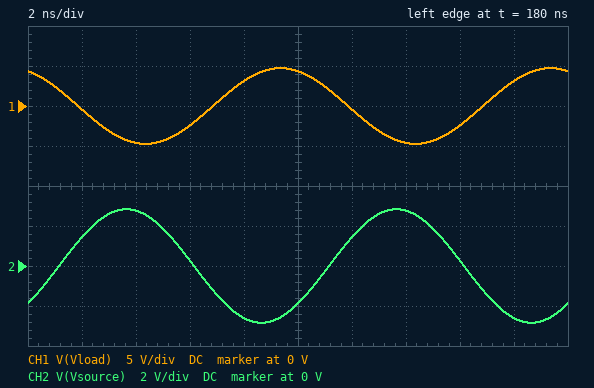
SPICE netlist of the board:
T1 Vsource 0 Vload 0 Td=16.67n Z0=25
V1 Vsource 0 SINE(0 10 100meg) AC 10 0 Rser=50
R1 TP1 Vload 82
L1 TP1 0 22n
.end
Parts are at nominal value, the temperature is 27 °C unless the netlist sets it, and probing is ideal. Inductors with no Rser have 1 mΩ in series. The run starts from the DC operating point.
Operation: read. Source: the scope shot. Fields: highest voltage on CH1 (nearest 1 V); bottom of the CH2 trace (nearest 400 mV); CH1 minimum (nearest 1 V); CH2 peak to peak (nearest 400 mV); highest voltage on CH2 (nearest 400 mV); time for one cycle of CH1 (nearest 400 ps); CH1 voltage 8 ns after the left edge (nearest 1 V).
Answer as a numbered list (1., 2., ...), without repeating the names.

1. 5 V
2. -2.8 V
3. -5 V
4. 5.6 V
5. 2.8 V
6. 10.0 ns
7. 3 V
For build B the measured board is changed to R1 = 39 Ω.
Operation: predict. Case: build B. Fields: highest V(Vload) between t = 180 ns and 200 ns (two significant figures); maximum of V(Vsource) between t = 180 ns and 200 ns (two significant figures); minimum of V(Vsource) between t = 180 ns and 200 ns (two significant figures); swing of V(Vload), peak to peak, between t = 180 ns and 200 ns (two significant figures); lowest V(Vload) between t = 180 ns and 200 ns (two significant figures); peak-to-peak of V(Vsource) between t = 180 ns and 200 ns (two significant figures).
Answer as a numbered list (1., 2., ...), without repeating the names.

1. 4.2 V
2. 3.5 V
3. -3.5 V
4. 8.4 V
5. -4.2 V
6. 7.0 V
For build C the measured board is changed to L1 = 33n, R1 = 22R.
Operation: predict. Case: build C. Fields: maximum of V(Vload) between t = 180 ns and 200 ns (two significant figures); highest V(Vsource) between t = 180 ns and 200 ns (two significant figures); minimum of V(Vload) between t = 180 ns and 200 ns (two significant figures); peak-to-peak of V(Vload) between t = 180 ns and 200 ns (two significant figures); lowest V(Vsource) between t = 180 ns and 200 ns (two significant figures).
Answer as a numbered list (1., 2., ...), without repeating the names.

1. 4.3 V
2. 4.8 V
3. -4.3 V
4. 8.6 V
5. -4.8 V
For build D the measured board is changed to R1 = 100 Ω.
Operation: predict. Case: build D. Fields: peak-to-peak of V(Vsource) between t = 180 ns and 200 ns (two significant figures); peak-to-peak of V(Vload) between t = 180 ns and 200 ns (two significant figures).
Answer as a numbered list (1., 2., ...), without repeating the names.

1. 5.5 V
2. 9.7 V
